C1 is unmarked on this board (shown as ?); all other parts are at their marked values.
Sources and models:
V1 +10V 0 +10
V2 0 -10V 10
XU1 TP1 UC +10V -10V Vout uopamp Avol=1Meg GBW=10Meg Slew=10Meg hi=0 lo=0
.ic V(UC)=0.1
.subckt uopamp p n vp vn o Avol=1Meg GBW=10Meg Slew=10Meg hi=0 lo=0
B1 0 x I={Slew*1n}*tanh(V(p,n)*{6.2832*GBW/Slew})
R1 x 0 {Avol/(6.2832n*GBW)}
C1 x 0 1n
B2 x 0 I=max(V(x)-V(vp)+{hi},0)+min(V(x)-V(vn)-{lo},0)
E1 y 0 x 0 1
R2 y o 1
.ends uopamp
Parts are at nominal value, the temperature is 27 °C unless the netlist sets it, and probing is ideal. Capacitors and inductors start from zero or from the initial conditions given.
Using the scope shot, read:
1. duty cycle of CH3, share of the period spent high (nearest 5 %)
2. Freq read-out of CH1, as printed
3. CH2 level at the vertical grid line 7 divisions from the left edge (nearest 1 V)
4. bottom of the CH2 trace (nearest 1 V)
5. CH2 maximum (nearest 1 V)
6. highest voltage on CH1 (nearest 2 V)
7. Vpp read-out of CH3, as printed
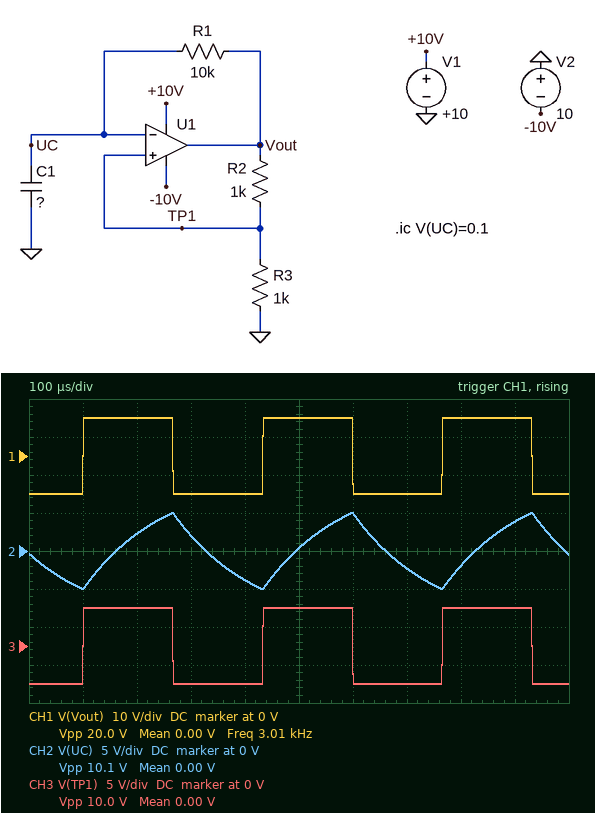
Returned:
50 %
3.01 kHz
-2 V
-5 V
5 V
10 V
10.0 V
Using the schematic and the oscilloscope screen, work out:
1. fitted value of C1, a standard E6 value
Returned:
15 nF
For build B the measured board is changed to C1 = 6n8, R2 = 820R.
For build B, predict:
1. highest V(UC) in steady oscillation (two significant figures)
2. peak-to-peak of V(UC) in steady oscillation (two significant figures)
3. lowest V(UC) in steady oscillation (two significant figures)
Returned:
5.5 V
11 V
-5.5 V
